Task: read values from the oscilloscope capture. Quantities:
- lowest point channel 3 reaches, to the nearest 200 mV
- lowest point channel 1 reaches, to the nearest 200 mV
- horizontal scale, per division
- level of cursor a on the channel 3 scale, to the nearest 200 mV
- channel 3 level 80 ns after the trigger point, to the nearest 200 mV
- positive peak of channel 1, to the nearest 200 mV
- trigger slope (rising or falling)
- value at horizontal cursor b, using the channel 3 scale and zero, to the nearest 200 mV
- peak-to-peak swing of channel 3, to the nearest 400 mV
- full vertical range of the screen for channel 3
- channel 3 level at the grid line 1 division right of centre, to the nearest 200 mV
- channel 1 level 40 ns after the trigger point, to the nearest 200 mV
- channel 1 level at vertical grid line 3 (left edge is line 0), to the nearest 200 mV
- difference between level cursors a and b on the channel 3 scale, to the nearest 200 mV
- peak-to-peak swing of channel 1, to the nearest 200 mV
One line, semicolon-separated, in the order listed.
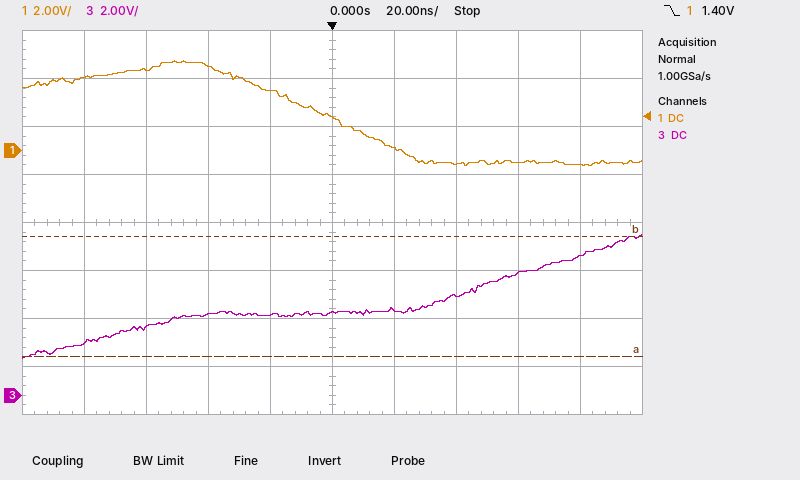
1.6 V; -600 mV; 20 ns; 1.6 V; 5.8 V; 3.8 V; falling; 6.6 V; 5.2 V; 16 V; 3.6 V; -600 mV; 3.6 V; 5.0 V; 4.4 V
